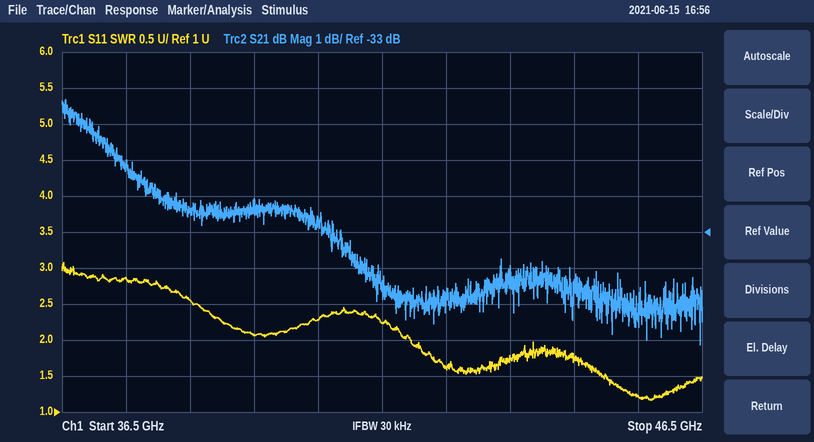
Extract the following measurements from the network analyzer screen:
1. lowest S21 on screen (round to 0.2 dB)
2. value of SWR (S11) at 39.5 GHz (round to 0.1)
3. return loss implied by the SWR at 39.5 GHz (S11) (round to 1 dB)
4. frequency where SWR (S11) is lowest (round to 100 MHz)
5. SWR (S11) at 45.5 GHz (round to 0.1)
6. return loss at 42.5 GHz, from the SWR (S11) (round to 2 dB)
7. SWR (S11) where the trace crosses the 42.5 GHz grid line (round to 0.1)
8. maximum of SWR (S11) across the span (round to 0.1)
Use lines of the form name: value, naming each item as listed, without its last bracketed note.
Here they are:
lowest S21 on screen: -36.2 dB
value of SWR (S11) at 39.5 GHz: 2.1
return loss implied by the SWR at 39.5 GHz (S11): 9 dB
frequency where SWR (S11) is lowest: 45.7 GHz
SWR (S11) at 45.5 GHz: 1.2
return loss at 42.5 GHz, from the SWR (S11): 12 dB
SWR (S11) where the trace crosses the 42.5 GHz grid line: 1.6
maximum of SWR (S11) across the span: 3.1
